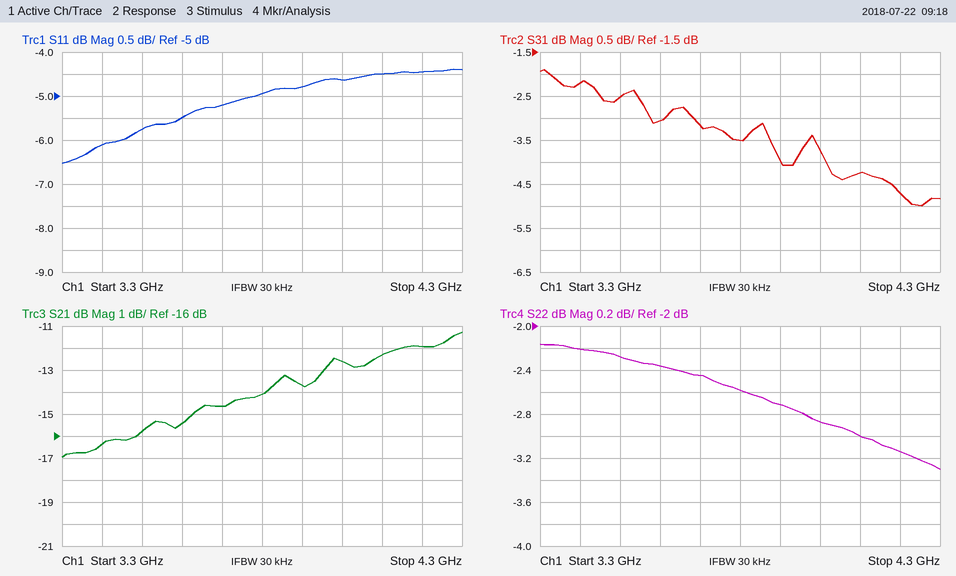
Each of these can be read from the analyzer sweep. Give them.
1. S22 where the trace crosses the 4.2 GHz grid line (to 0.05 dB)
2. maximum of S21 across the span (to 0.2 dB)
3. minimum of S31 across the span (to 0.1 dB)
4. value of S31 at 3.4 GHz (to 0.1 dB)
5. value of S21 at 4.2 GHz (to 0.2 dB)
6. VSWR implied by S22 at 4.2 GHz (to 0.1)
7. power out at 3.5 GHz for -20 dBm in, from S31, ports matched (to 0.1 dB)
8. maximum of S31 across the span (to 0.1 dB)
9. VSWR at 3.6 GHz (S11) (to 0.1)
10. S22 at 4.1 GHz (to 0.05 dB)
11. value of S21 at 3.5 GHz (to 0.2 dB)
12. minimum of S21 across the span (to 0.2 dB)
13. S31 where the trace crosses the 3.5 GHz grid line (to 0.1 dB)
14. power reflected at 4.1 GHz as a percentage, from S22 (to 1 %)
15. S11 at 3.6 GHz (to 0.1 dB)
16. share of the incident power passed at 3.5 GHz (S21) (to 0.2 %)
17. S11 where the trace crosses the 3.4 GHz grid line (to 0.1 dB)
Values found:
-3.15 dB
-11.2 dB
-5.0 dB
-2.2 dB
-12.0 dB
5.6
-22.5 dBm
-1.9 dB
3.3
-3.00 dB
-15.8 dB
-17.0 dB
-2.5 dB
50 %
-5.5 dB
2.6 %
-6.1 dB
